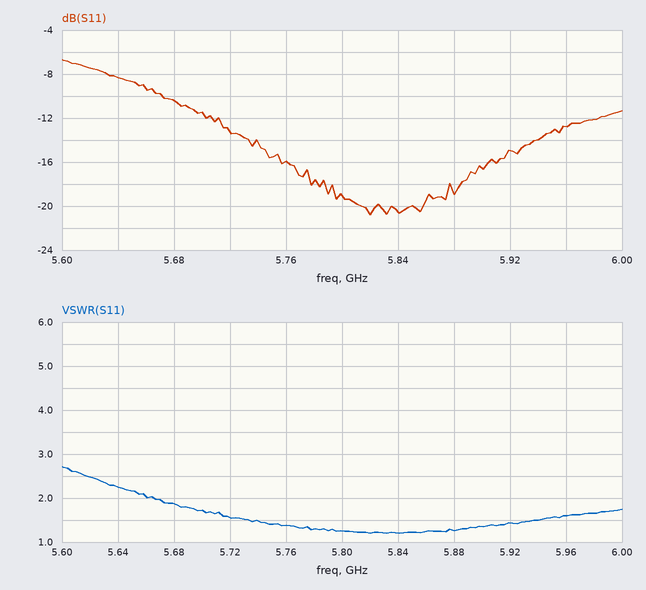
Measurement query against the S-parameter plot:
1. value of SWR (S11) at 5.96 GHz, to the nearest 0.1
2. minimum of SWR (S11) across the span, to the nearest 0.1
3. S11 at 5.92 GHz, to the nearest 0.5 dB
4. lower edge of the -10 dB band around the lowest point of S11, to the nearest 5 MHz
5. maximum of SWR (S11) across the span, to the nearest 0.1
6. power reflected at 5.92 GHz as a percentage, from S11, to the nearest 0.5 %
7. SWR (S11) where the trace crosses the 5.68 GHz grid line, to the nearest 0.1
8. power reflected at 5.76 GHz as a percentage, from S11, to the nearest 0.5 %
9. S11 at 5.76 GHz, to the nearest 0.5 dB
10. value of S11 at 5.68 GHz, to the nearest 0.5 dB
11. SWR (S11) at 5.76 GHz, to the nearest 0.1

1.6
1.2
-15.0 dB
5.670 GHz
2.7
3.0 %
1.9
2.5 %
-16.0 dB
-10.5 dB
1.4
